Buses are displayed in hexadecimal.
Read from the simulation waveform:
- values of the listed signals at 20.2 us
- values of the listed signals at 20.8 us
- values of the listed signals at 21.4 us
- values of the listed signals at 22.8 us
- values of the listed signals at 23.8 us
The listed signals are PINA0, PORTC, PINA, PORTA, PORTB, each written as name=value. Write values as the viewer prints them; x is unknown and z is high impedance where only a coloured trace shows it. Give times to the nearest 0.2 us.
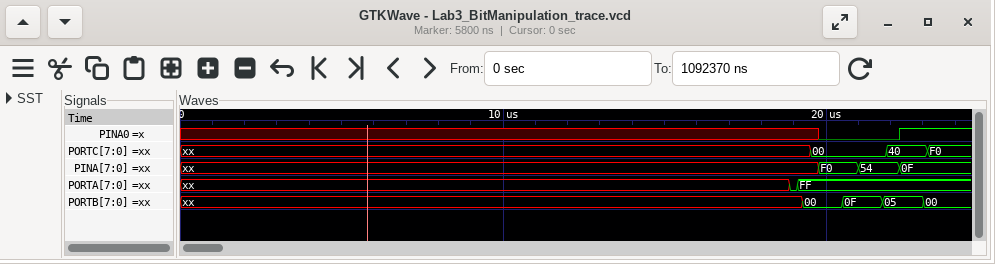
PINA0=0, PORTC=00, PINA=F0, PORTA=FF, PORTB=00
PINA0=0, PORTC=00, PINA=F0, PORTA=FF, PORTB=0F
PINA0=0, PORTC=00, PINA=54, PORTA=FF, PORTB=0F
PINA0=1, PORTC=40, PINA=0F, PORTA=FF, PORTB=05
PINA0=1, PORTC=F0, PINA=0F, PORTA=FF, PORTB=00
